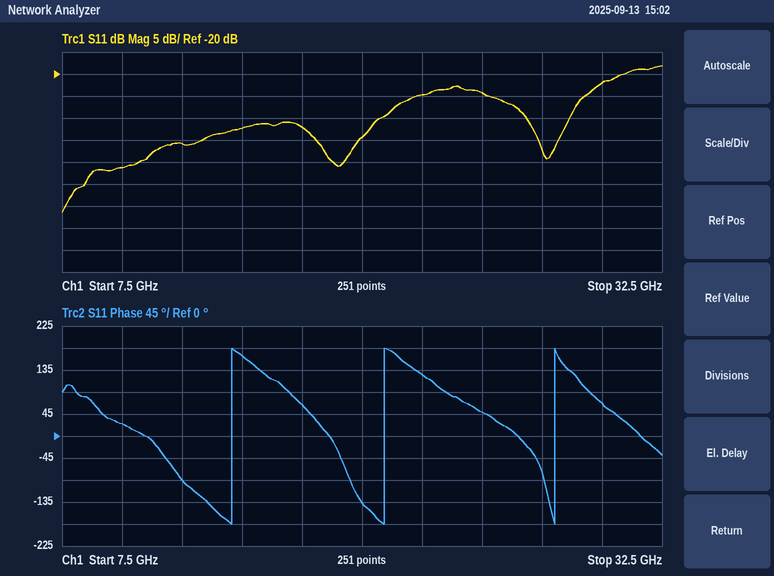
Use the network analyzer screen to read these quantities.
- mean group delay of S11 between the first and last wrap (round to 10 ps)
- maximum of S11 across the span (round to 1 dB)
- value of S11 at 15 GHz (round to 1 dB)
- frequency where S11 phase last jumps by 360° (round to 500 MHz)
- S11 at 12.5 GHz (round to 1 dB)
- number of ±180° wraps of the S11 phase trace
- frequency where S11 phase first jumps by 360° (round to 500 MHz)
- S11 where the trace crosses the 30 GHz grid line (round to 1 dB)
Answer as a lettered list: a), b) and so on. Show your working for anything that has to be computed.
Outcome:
a) 2 cycles / (28.0 GHz − 14.5 GHz) ≈ 148 ps, so 150 ps to the nearest 10 ps
b) -18 dB
c) -32 dB
d) 28.0 GHz
e) -36 dB
f) 3
g) 14.5 GHz
h) -22 dB
